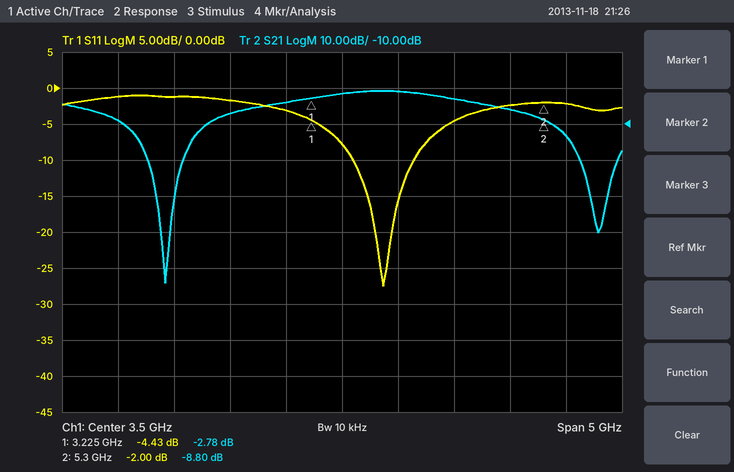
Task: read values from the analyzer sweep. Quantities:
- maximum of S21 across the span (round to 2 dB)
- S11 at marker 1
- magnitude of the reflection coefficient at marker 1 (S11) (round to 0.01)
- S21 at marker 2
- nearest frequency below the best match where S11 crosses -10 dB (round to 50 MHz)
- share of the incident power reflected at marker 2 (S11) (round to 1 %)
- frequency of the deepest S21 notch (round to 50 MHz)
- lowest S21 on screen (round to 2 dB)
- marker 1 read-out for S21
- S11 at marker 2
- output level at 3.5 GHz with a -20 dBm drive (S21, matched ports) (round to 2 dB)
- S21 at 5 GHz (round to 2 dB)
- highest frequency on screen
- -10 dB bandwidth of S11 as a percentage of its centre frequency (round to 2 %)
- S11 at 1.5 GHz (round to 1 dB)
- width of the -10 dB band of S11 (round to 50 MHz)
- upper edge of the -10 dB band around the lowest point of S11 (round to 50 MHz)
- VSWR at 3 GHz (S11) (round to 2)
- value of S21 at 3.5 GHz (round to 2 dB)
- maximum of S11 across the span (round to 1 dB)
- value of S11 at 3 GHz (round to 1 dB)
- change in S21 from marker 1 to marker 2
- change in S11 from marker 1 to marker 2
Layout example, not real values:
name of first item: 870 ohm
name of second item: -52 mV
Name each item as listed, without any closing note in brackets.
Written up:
maximum of S21 across the span: 0 dB
S11 at marker 1: -4.43 dB
magnitude of the reflection coefficient at marker 1 (S11): 0.60
S21 at marker 2: -8.80 dB
nearest frequency below the best match where S11 crosses -10 dB: 3.60 GHz
share of the incident power reflected at marker 2 (S11): 63 %
frequency of the deepest S21 notch: 1.90 GHz
lowest S21 on screen: -54 dB
marker 1 read-out for S21: -2.78 dB
S11 at marker 2: -2.00 dB
output level at 3.5 GHz with a -20 dBm drive (S21, matched ports): -22 dBm
S21 at 5 GHz: -6 dB
highest frequency on screen: 6 GHz
-10 dB bandwidth of S11 as a percentage of its centre frequency: 14 %
S11 at 1.5 GHz: -1 dB
width of the -10 dB band of S11: 550 MHz
upper edge of the -10 dB band around the lowest point of S11: 4.15 GHz
VSWR at 3 GHz (S11): 6
value of S21 at 3.5 GHz: -2 dB
maximum of S11 across the span: -1 dB
value of S11 at 3 GHz: -3 dB
change in S21 from marker 1 to marker 2: -6.02 dB
change in S11 from marker 1 to marker 2: 2.43 dB
